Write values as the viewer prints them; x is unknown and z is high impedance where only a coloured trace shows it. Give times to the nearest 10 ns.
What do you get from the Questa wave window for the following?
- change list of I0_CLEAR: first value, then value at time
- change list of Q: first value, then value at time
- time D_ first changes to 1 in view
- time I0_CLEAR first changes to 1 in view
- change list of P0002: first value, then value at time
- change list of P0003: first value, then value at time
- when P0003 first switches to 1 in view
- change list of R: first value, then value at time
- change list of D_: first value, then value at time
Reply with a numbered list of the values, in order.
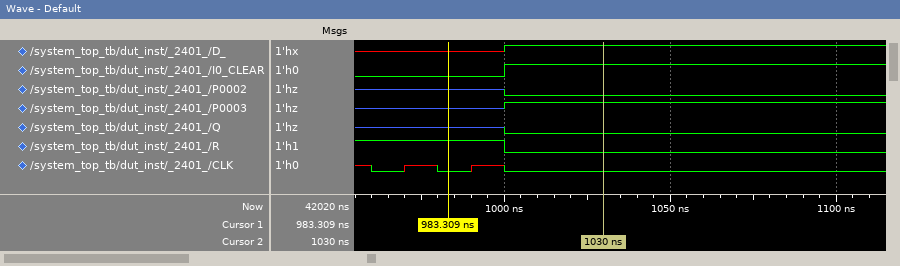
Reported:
1. 0, 1 at 1000 ns
2. z, 0 at 1000 ns
3. 1000 ns
4. 1000 ns
5. z, 0 at 1000 ns
6. z, 1 at 1000 ns
7. 1000 ns
8. 1, 0 at 1000 ns
9. x, 1 at 1000 ns
